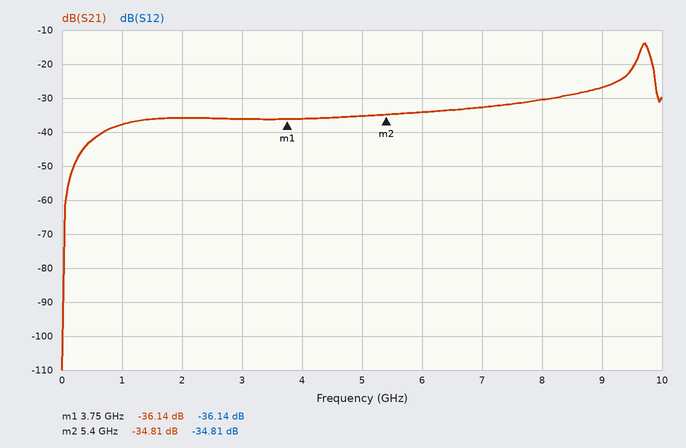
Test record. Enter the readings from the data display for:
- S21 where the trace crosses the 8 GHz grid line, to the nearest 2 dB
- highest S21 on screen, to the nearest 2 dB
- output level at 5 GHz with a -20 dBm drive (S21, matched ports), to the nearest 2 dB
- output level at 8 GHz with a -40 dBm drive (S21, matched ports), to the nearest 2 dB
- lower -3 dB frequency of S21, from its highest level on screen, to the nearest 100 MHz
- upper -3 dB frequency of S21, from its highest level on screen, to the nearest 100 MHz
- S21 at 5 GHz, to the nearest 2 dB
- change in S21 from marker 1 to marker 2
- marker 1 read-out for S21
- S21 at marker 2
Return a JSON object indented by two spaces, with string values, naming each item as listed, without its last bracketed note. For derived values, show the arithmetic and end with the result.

{
  "S21 where the trace crosses the 8 GHz grid line, to the nearest 2 dB": "-30 dB",
  "highest S21 on screen, to the nearest 2 dB": "-14 dB",
  "output level at 5 GHz with a -20 dBm drive (S21, matched ports), to the nearest 2 dB": "-20 dBm + (-36 dB) = -56 dBm",
  "output level at 8 GHz with a -40 dBm drive (S21, matched ports), to the nearest 2 dB": "-40 dBm + (-30 dB) = -70 dBm",
  "lower -3 dB frequency of S21, from its highest level on screen, to the nearest 100 MHz": "9.6 GHz",
  "upper -3 dB frequency of S21, from its highest level on screen, to the nearest 100 MHz": "9.8 GHz",
  "S21 at 5 GHz, to the nearest 2 dB": "-36 dB",
  "change in S21 from marker 1 to marker 2": "-34.81 − (-36.14) = 1.33 dB",
  "marker 1 read-out for S21": "-36.14 dB",
  "S21 at marker 2": "-34.81 dB"
}
